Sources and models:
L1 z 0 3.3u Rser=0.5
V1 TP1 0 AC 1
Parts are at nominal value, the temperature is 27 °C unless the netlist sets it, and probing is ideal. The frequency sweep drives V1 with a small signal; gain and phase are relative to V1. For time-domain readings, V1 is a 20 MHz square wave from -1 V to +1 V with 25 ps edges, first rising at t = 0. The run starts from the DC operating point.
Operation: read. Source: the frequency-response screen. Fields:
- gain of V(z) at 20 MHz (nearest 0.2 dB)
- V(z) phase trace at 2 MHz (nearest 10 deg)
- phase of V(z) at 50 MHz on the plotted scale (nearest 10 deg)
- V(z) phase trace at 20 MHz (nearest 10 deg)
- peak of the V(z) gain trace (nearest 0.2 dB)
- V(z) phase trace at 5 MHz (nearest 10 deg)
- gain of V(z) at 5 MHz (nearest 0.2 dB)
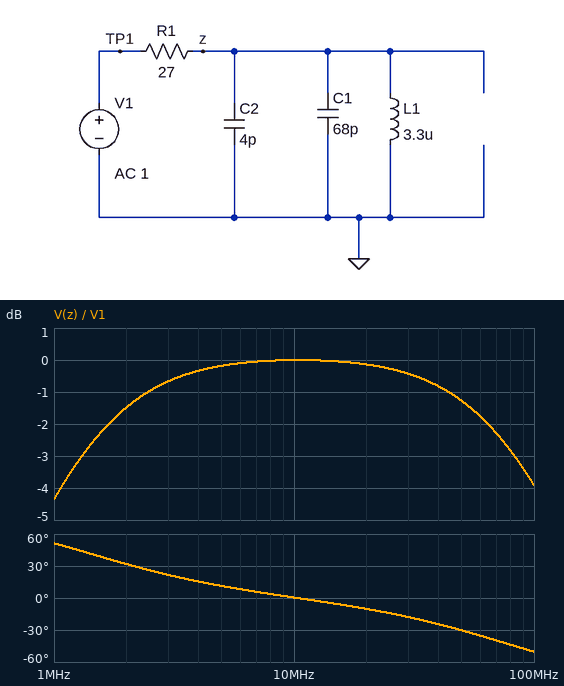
-0.2 dB
30 deg
-30 deg
-10 deg
0 dB
10 deg
-0.2 dB
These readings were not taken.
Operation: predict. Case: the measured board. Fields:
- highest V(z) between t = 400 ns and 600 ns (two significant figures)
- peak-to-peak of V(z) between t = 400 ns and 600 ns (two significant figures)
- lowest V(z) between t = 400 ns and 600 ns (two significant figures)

1.1 V
2.1 V
-1.0 V
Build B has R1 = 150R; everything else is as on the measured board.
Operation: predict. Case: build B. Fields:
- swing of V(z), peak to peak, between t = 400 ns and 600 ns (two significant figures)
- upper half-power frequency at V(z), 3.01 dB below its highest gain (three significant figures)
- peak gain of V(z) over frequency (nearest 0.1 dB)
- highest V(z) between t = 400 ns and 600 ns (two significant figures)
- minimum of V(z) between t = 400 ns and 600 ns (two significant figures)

1.7 V
20.1 MHz
0 dB
860 mV
-860 mV
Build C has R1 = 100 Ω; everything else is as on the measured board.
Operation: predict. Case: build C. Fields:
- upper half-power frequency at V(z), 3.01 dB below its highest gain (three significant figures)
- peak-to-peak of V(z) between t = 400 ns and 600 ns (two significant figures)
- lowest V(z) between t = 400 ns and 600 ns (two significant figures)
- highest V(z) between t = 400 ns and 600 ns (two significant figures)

26.2 MHz
1.9 V
-950 mV
950 mV
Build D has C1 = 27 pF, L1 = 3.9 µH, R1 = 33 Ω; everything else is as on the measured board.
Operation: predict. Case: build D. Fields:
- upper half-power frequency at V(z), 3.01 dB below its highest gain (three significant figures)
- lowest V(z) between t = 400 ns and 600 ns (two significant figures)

157 MHz
-1.1 V
